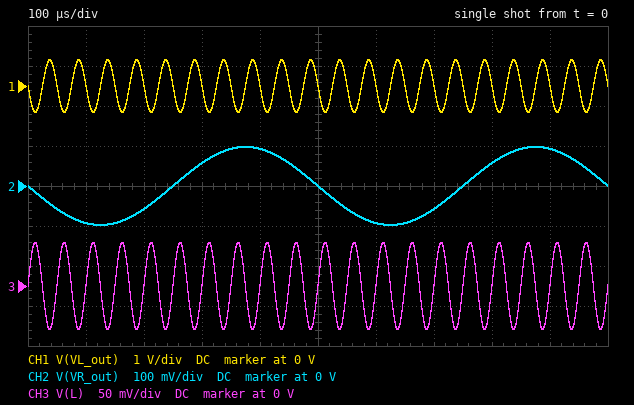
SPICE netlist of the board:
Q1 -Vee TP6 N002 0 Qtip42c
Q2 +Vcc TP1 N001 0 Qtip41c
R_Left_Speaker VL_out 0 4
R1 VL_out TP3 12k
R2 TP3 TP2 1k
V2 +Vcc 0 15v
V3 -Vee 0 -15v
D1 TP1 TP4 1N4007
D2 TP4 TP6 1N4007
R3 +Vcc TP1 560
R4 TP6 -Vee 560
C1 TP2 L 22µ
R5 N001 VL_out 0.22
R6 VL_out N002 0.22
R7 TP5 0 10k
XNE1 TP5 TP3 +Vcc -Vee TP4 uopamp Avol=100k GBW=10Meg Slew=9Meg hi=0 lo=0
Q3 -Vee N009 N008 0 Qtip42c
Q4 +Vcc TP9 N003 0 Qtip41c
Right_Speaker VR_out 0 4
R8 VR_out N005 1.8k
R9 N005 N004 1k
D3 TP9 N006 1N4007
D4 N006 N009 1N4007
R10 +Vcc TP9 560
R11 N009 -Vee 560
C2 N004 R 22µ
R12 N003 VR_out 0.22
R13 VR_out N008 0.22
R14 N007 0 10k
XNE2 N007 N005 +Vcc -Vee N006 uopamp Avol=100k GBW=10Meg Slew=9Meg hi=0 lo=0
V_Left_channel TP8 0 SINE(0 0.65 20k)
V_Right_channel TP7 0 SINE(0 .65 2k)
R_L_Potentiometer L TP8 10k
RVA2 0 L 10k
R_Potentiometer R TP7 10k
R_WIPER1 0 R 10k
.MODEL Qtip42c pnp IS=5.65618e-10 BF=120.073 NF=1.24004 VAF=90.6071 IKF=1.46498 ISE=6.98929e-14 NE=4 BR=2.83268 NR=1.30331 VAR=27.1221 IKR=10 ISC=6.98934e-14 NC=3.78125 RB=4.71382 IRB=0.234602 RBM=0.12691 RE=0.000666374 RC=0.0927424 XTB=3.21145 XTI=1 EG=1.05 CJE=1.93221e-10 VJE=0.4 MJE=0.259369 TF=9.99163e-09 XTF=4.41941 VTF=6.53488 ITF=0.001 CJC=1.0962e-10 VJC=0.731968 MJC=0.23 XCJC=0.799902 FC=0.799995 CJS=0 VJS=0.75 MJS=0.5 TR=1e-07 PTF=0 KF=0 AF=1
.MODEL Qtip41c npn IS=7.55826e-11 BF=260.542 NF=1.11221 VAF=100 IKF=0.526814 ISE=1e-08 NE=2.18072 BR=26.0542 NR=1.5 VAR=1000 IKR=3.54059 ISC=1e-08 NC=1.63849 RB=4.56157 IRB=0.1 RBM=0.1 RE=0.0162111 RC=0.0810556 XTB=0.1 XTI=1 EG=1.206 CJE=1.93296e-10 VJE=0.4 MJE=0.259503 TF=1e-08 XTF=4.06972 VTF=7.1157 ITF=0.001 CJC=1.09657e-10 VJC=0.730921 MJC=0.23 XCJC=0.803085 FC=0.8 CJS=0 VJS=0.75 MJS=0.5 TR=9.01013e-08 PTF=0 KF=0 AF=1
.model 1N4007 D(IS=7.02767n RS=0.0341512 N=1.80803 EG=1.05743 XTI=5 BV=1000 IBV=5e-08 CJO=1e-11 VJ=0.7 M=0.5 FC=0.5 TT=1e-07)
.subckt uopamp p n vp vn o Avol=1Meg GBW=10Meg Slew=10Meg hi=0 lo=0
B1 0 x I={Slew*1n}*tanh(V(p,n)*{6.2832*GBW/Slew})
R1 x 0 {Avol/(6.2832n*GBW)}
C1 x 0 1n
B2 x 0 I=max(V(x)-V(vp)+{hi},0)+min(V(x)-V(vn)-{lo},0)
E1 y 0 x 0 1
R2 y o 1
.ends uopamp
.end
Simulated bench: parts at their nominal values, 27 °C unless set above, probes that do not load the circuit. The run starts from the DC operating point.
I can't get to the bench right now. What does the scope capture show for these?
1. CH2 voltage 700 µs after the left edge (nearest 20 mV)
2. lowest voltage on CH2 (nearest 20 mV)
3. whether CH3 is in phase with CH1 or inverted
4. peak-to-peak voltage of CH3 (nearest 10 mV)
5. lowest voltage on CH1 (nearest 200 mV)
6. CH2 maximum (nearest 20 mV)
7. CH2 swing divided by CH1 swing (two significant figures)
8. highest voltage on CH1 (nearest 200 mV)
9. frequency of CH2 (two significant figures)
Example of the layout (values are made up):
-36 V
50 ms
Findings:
-60 mV
-100 mV
inverted
110 mV
-600 mV
100 mV
0.15
600 mV
2.0 kHz
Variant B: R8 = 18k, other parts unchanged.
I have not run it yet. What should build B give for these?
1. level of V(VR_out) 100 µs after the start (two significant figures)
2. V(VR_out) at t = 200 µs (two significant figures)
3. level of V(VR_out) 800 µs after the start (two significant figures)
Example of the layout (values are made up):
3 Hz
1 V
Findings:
-930 mV
-570 mV
570 mV
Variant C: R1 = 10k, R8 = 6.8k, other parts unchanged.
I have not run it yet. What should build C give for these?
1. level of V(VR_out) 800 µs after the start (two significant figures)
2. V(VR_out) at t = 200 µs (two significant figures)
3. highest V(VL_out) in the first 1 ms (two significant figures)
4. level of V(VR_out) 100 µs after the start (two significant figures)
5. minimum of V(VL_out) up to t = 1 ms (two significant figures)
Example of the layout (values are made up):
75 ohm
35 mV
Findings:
220 mV
-220 mV
540 mV
-350 mV
-540 mV
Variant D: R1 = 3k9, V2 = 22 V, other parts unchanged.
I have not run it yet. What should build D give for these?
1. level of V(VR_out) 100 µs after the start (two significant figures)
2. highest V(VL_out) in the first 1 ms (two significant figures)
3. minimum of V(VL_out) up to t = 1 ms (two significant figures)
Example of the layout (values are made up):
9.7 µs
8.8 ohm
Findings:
-93 mV
210 mV
-210 mV
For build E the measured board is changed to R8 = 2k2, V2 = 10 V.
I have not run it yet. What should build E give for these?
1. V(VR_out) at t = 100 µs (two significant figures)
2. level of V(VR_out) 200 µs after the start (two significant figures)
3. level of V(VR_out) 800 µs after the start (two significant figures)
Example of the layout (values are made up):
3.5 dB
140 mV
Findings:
-110 mV
-70 mV
70 mV
